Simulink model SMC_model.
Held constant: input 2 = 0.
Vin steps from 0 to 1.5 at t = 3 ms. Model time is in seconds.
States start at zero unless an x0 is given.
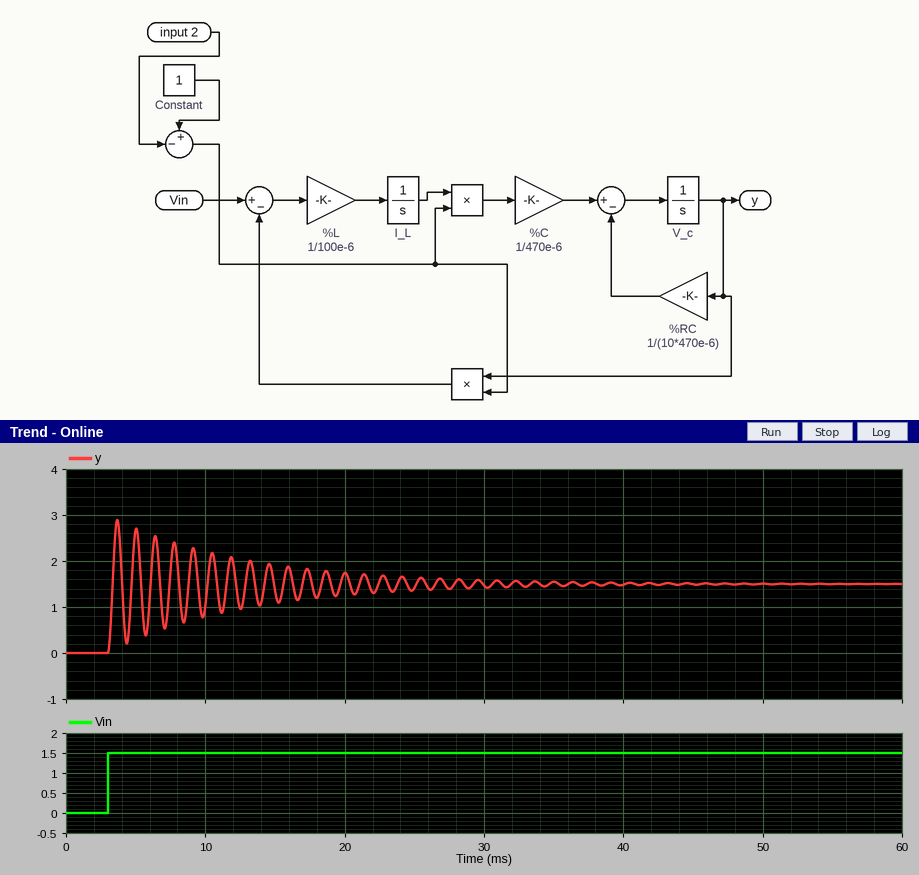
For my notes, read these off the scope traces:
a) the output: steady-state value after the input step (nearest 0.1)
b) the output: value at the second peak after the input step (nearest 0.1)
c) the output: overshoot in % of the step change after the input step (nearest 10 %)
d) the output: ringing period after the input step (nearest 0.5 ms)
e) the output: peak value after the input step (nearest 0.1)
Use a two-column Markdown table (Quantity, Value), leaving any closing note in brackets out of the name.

| Quantity | Value |
|---|---|
| the output: steady-state value after the input step | 1.5 |
| the output: value at the second peak after the input step | 2.7 |
| the output: overshoot in % of the step change after the input step | 90 % |
| the output: ringing period after the input step | 1.5 ms |
| the output: peak value after the input step | 2.9 |
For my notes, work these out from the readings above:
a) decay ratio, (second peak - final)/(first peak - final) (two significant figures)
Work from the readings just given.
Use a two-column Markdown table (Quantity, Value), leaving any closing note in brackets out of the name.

| Quantity | Value |
|---|---|
| decay ratio, (second peak - final)/(first peak - final) | 0.86 |
